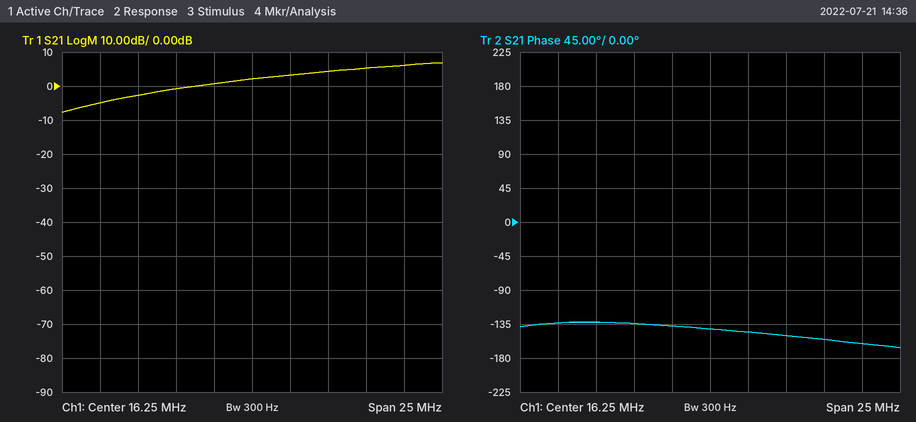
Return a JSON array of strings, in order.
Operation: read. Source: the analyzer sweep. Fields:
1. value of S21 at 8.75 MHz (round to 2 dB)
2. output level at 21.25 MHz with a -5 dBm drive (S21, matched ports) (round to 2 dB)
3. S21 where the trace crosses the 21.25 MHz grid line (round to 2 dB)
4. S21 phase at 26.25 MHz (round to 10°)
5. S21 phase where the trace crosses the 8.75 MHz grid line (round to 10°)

["-2 dB", "0 dBm", "4 dB", "-160°", "-130°"]
